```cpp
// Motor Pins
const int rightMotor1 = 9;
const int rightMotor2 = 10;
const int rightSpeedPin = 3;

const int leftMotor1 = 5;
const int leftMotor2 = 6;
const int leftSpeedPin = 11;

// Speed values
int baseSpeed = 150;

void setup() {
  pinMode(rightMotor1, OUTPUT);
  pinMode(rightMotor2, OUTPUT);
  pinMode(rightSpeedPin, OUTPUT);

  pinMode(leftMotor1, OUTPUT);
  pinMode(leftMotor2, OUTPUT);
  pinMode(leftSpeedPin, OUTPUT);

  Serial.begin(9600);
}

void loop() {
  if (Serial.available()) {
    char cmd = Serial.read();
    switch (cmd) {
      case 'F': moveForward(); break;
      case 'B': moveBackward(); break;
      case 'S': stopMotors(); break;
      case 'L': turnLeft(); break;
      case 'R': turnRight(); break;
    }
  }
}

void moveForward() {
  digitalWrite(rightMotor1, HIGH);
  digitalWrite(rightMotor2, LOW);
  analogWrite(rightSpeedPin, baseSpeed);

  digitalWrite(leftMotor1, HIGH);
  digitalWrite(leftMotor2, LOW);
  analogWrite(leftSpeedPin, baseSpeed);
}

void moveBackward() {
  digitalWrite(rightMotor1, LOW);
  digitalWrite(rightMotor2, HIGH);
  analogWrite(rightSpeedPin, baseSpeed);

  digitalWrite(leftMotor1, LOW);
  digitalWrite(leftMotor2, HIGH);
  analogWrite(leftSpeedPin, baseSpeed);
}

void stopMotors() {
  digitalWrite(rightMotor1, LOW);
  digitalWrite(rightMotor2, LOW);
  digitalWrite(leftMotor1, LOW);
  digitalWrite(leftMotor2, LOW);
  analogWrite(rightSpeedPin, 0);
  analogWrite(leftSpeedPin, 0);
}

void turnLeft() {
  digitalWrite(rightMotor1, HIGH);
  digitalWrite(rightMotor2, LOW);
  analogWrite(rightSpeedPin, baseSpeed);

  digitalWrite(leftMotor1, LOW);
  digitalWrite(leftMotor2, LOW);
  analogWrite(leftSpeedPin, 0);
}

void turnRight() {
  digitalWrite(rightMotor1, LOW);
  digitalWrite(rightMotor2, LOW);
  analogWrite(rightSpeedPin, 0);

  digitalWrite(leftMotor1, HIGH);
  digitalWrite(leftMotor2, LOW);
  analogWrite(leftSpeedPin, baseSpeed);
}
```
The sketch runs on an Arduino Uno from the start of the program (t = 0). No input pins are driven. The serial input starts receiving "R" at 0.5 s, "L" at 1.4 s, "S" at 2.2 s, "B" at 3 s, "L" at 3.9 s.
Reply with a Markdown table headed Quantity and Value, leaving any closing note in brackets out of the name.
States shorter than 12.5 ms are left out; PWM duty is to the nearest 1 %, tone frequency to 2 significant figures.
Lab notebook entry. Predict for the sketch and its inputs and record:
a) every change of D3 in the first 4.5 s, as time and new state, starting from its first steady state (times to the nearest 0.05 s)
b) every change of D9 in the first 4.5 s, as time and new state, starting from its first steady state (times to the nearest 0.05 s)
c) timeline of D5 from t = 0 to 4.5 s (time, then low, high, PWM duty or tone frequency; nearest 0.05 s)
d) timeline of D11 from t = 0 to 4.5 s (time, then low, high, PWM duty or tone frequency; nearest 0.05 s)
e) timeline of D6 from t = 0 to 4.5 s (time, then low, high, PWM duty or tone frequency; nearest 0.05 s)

| Quantity | Value |
|---|---|
| every change of D3 in the first 4.5 s, as time and new state, starting from its first steady state | 0 s low; 1.4 s PWM 59 %; 2.2 s low; 3 s PWM 59 % |
| every change of D9 in the first 4.5 s, as time and new state, starting from its first steady state | 0 s low; 1.4 s high; 2.2 s low; 3.9 s high |
| timeline of D5 from t = 0 to 4.5 s | 0 s low; 0.5 s high; 1.4 s low |
| timeline of D11 from t = 0 to 4.5 s | 0 s low; 0.5 s PWM 59 %; 1.4 s low; 3 s PWM 59 %; 3.9 s low |
| timeline of D6 from t = 0 to 4.5 s | 0 s low; 3 s high; 3.9 s low |
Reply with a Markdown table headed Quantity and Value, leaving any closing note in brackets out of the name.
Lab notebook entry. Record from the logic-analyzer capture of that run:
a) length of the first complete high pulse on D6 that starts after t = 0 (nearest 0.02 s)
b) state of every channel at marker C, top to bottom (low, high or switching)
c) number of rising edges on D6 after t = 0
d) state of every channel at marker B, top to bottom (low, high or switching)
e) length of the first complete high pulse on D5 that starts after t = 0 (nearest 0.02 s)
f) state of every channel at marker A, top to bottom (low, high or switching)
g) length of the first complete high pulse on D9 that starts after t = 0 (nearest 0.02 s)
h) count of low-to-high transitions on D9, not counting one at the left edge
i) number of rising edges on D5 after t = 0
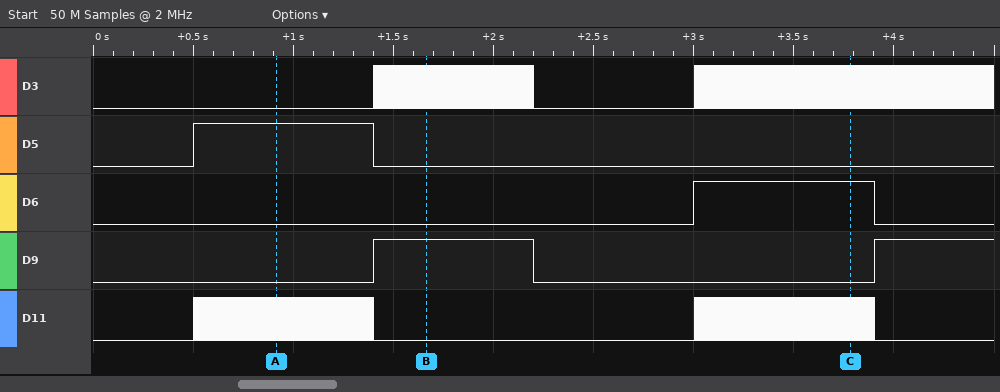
| Quantity | Value |
|---|---|
| length of the first complete high pulse on D6 that starts after t = 0 | 0.90 s |
| state of every channel at marker C, top to bottom | D3 switching, D5 low, D6 high, D9 low, D11 switching |
| number of rising edges on D6 after t = 0 | 1 |
| state of every channel at marker B, top to bottom | D3 switching, D5 low, D6 low, D9 high, D11 low |
| length of the first complete high pulse on D5 that starts after t = 0 | 0.90 s |
| state of every channel at marker A, top to bottom | D3 low, D5 high, D6 low, D9 low, D11 switching |
| length of the first complete high pulse on D9 that starts after t = 0 | 0.80 s |
| count of low-to-high transitions on D9, not counting one at the left edge | 2 |
| number of rising edges on D5 after t = 0 | 1 |
